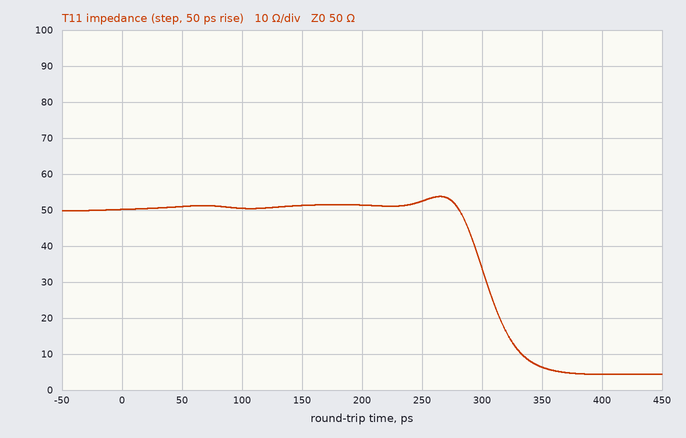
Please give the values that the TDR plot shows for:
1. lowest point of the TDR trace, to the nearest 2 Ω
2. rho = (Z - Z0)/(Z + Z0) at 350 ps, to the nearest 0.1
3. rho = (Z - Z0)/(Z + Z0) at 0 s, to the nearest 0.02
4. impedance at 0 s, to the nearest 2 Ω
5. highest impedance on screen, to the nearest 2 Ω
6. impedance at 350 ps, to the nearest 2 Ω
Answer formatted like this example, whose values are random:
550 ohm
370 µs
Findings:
4 Ω
-0.8
0.00
50 Ω
54 Ω
6 Ω
